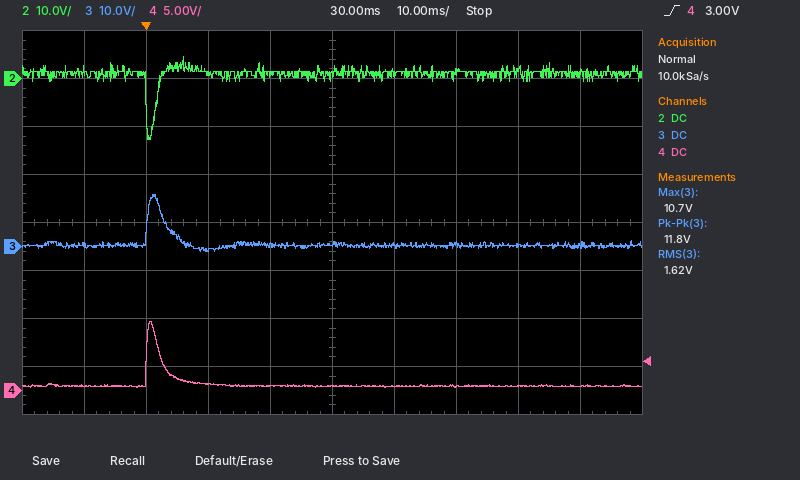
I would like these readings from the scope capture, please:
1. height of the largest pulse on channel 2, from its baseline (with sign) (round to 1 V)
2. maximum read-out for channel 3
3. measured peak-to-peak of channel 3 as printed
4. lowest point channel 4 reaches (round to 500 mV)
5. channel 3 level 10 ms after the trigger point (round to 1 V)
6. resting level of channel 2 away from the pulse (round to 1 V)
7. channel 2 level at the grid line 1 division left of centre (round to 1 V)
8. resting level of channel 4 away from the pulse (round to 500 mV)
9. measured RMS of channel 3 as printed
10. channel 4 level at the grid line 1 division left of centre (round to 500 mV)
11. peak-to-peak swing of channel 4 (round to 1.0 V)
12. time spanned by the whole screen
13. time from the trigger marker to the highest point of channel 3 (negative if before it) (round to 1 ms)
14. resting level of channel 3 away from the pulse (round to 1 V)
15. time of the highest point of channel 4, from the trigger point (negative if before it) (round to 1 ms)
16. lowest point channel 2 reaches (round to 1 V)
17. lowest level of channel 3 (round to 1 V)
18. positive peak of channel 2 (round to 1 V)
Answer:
-14 V
10.7 V
11.8 V
500 mV
-1 V
1 V
1 V
500 mV
1.62 V
500 mV
7.0 V
100 ms
+1 ms
0 V
+1 ms
-13 V
-1 V
5 V
